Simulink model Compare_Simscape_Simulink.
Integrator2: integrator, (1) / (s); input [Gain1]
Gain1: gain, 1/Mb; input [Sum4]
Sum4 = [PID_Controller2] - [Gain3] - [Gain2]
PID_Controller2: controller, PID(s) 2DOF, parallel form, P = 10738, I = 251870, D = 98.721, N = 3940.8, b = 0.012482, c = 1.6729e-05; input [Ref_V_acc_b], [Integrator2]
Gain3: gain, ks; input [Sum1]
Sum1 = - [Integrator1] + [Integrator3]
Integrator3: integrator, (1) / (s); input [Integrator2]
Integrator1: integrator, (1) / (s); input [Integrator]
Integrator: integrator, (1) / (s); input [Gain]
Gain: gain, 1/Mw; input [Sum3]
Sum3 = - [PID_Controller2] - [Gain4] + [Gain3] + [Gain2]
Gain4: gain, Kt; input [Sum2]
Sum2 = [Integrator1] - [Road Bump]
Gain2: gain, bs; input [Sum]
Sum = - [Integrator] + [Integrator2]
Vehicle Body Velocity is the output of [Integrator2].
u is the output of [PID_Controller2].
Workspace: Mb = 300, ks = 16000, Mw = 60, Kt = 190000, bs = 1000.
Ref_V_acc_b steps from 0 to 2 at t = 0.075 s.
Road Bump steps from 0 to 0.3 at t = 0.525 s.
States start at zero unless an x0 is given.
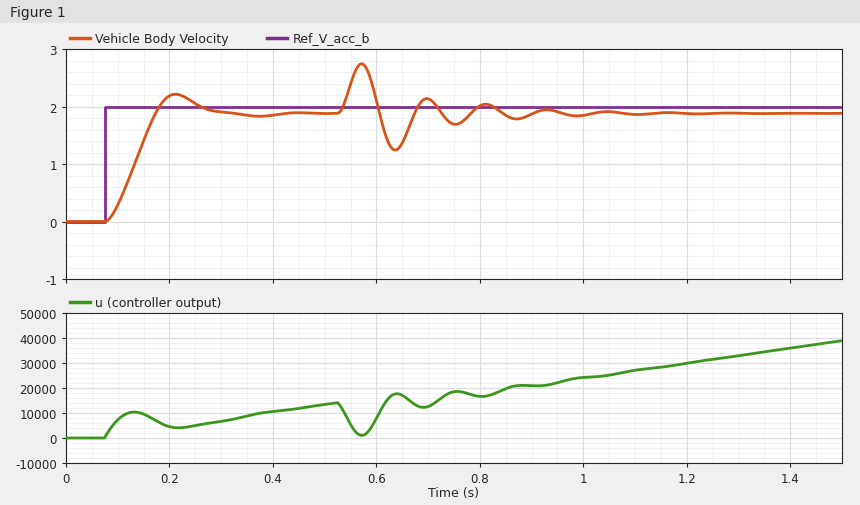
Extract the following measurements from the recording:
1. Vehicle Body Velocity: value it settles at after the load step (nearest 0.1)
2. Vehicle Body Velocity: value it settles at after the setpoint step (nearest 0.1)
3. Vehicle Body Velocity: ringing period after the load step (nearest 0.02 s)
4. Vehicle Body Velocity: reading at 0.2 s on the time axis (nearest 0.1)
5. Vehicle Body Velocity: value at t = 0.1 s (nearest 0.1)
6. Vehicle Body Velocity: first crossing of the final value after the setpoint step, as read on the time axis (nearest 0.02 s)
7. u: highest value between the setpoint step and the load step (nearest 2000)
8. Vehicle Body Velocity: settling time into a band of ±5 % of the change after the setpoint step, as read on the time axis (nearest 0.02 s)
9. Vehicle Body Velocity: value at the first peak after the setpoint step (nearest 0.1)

1.9
1.9
0.12 s
2.2
0.3
0.18 s
14000
0.26 s
2.2
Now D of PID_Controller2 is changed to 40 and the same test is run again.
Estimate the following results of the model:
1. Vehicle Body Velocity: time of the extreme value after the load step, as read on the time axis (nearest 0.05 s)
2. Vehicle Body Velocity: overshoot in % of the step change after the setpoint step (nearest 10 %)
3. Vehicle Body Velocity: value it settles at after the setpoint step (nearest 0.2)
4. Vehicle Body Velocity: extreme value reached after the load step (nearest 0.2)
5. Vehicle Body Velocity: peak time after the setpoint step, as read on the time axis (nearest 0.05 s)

0.55 s
20 %
1.8
2.8
0.20 s
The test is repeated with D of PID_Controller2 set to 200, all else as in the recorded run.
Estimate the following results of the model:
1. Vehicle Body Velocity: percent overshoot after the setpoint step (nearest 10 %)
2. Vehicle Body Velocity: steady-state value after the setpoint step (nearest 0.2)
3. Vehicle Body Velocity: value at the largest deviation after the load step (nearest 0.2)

20 %
1.8
2.6
